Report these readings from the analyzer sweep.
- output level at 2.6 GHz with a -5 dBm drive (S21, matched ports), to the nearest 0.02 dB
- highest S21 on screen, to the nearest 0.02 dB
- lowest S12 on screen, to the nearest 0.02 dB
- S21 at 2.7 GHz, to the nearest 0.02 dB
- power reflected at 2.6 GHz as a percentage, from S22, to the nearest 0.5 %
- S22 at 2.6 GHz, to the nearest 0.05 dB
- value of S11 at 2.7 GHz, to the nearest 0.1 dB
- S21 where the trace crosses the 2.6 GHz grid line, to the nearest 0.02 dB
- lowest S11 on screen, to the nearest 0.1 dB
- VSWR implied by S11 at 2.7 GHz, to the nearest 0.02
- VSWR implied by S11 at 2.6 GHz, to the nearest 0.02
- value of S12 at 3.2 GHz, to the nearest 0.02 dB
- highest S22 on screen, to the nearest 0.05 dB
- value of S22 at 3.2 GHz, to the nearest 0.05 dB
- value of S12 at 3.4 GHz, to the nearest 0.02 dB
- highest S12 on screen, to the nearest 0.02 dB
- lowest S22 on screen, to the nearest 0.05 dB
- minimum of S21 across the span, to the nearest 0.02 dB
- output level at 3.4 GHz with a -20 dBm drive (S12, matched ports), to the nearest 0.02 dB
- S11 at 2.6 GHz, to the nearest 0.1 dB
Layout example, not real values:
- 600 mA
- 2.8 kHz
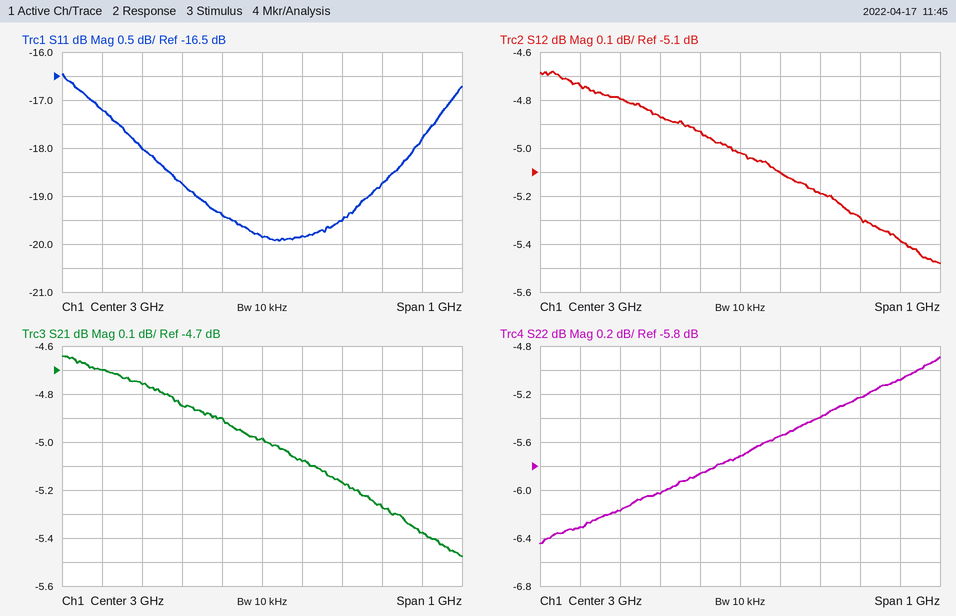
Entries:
- -9.70 dBm
- -4.64 dB
- -5.48 dB
- -4.76 dB
- 23.5 %
- -6.30 dB
- -18.0 dB
- -4.70 dB
- -19.9 dB
- 1.28
- 1.32
- -5.18 dB
- -4.90 dB
- -5.40 dB
- -5.38 dB
- -4.68 dB
- -6.45 dB
- -5.48 dB
- -25.38 dBm
- -17.2 dB
